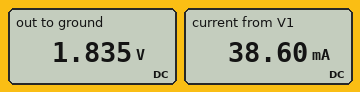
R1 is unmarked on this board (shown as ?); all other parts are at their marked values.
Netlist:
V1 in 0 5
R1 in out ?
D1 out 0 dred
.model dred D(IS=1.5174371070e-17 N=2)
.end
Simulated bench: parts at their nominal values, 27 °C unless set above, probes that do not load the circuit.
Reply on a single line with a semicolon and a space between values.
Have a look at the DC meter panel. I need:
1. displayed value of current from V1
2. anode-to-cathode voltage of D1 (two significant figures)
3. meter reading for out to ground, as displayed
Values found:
38.60 mA; 1.8 V; 1.835 V
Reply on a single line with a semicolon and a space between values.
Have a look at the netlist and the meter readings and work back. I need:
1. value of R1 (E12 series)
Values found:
82 Ω
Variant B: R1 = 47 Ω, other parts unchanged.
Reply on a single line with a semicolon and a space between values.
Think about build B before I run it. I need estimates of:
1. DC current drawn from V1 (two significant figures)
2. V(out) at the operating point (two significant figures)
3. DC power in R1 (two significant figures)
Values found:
67 mA; 1.9 V; 210 mW
